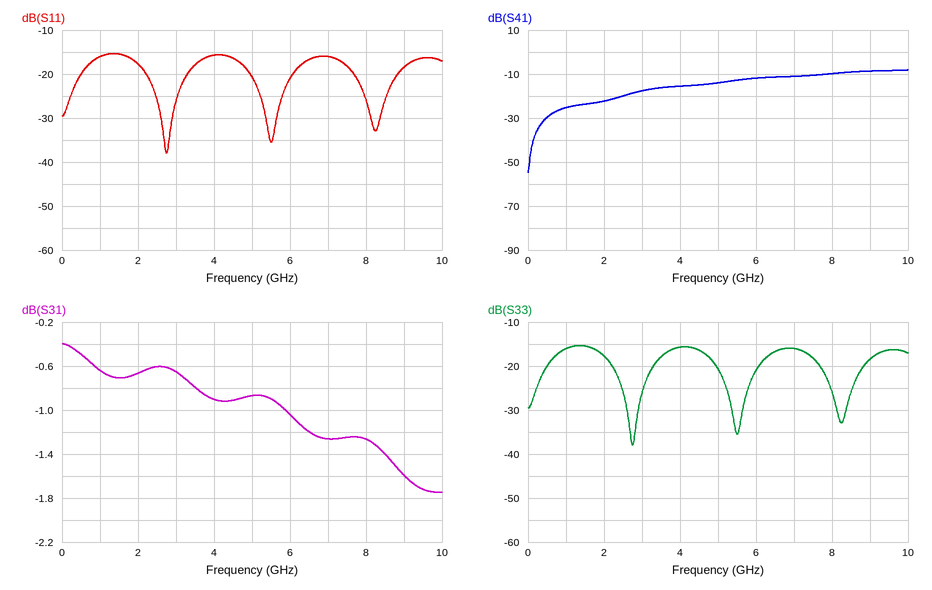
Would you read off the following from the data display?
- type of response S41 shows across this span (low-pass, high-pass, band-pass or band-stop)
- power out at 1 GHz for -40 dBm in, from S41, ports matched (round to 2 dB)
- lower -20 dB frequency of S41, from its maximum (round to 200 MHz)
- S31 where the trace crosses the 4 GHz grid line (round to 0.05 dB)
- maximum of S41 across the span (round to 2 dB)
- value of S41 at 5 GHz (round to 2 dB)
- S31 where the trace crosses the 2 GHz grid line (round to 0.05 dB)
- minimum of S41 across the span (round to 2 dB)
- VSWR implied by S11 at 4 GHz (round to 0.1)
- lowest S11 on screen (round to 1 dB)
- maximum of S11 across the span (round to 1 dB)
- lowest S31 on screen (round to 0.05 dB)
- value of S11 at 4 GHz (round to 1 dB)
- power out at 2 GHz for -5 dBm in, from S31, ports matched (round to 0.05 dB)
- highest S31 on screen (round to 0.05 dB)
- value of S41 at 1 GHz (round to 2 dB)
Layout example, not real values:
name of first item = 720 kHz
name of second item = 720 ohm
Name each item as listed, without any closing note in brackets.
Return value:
type of response S41 shows across this span = high-pass
power out at 1 GHz for -40 dBm in, from S41, ports matched = -66 dBm
lower -20 dB frequency of S41, from its maximum = 600 MHz
S31 where the trace crosses the 4 GHz grid line = -0.90 dB
maximum of S41 across the span = -8 dB
value of S41 at 5 GHz = -14 dB
S31 where the trace crosses the 2 GHz grid line = -0.65 dB
minimum of S41 across the span = -54 dB
VSWR implied by S11 at 4 GHz = 1.4
lowest S11 on screen = -38 dB
maximum of S11 across the span = -15 dB
lowest S31 on screen = -1.75 dB
value of S11 at 4 GHz = -16 dB
power out at 2 GHz for -5 dBm in, from S31, ports matched = -5.65 dBm
highest S31 on screen = -0.40 dB
value of S41 at 1 GHz = -26 dB
